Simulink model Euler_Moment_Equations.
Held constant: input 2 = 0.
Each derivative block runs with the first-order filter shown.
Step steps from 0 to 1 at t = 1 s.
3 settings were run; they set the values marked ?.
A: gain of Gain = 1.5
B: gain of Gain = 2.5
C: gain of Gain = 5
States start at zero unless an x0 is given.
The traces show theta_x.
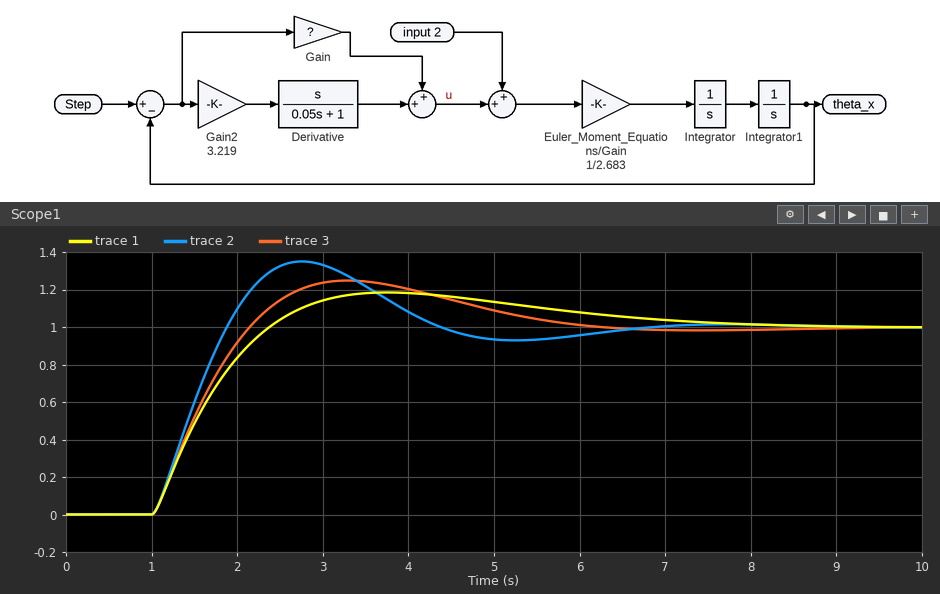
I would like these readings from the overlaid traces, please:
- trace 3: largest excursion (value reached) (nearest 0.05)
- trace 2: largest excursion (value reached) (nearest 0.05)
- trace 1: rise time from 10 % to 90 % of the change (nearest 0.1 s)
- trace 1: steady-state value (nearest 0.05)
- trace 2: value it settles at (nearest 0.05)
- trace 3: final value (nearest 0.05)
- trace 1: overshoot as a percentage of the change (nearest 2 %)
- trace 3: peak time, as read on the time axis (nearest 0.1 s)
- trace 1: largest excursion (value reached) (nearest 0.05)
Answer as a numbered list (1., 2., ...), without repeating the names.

1. 1.25
2. 1.35
3. 1.0 s
4. 1.00
5. 1.00
6. 1.00
7. 18 %
8. 3.3 s
9. 1.20
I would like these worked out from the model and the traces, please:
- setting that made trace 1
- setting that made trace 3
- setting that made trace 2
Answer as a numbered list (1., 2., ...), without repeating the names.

1. A
2. B
3. C
